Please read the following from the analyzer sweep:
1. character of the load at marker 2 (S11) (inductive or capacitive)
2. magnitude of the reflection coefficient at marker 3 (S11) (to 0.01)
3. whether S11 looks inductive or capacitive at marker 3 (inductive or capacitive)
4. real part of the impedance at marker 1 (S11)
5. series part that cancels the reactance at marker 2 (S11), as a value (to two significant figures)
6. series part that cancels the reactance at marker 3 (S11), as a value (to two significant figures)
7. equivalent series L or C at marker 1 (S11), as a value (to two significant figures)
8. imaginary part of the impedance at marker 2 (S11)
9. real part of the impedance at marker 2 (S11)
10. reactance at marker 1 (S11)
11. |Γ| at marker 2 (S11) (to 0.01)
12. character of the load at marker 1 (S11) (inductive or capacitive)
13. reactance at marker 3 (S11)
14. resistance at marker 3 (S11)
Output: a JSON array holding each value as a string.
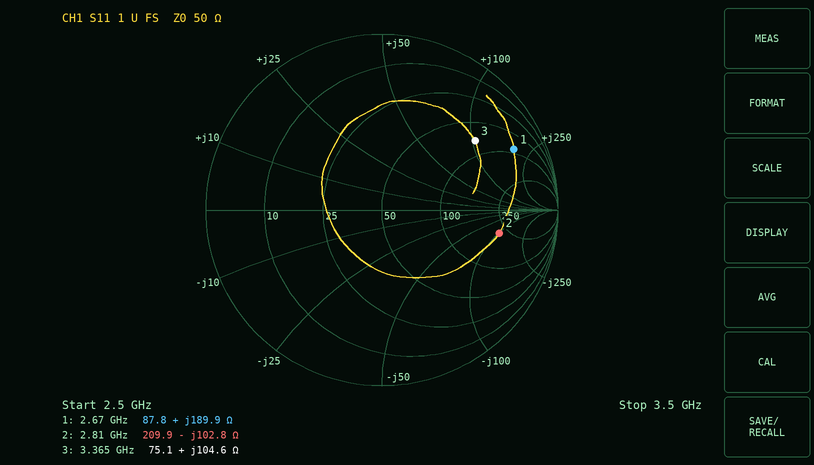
["capacitive", "0.66", "inductive", "87.8 Ω", "5.8 nH", "450 fF", "11 nH", "-102.8 Ω", "209.9 Ω", "+189.9 Ω", "0.68", "inductive", "+104.6 Ω", "75.1 Ω"]
